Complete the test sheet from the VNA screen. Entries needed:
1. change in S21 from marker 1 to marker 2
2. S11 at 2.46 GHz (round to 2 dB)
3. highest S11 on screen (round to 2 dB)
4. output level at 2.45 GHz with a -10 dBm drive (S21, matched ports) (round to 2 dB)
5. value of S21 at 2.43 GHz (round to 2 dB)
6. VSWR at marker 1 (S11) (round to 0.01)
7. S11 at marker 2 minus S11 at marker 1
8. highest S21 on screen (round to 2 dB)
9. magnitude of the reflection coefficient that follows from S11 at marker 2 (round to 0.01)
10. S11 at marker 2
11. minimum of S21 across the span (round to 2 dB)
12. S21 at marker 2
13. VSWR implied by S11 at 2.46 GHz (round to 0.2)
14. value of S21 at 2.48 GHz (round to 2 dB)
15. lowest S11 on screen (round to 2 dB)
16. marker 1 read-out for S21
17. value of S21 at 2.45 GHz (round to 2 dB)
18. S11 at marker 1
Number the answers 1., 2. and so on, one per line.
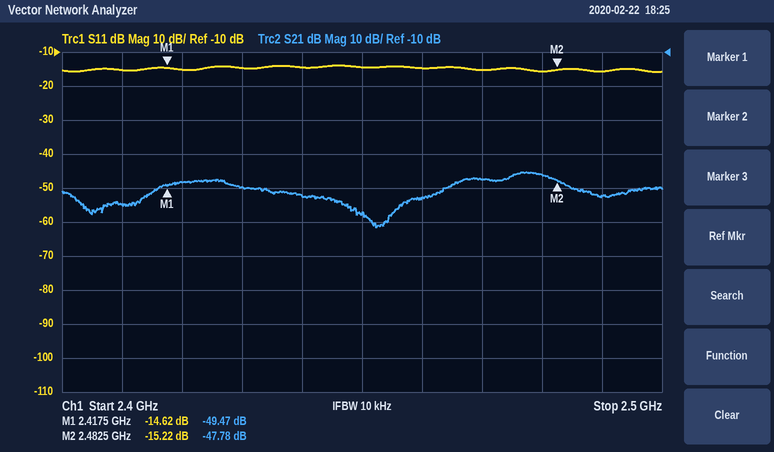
1. 1.69 dB
2. -14 dB
3. -14 dB
4. -68 dBm
5. -50 dB
6. 1.46
7. -0.60 dB
8. -46 dB
9. 0.17
10. -15.22 dB
11. -62 dB
12. -47.78 dB
13. 1.4
14. -46 dB
15. -16 dB
16. -49.47 dB
17. -58 dB
18. -14.62 dB
